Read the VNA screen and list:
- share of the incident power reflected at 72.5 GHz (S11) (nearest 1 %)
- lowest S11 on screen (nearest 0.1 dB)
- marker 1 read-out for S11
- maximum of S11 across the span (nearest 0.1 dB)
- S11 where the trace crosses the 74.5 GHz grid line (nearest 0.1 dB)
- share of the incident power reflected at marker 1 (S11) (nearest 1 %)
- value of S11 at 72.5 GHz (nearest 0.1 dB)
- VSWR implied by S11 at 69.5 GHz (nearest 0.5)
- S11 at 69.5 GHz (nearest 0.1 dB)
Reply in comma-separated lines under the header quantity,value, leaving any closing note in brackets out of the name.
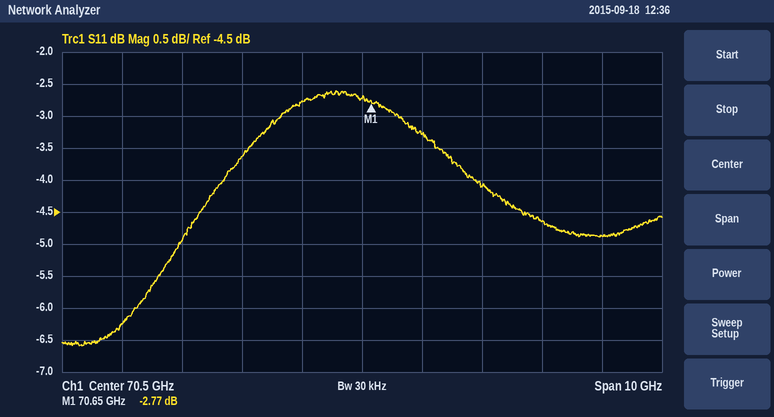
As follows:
quantity,value
share of the incident power reflected at 72.5 GHz (S11),39 %
lowest S11 on screen,-6.6 dB
marker 1 read-out for S11,-2.77 dB
maximum of S11 across the span,-2.6 dB
S11 where the trace crosses the 74.5 GHz grid line,-4.9 dB
share of the incident power reflected at marker 1 (S11),53 %
value of S11 at 72.5 GHz,-4.1 dB
VSWR implied by S11 at 69.5 GHz,6.5
S11 at 69.5 GHz,-2.8 dB
